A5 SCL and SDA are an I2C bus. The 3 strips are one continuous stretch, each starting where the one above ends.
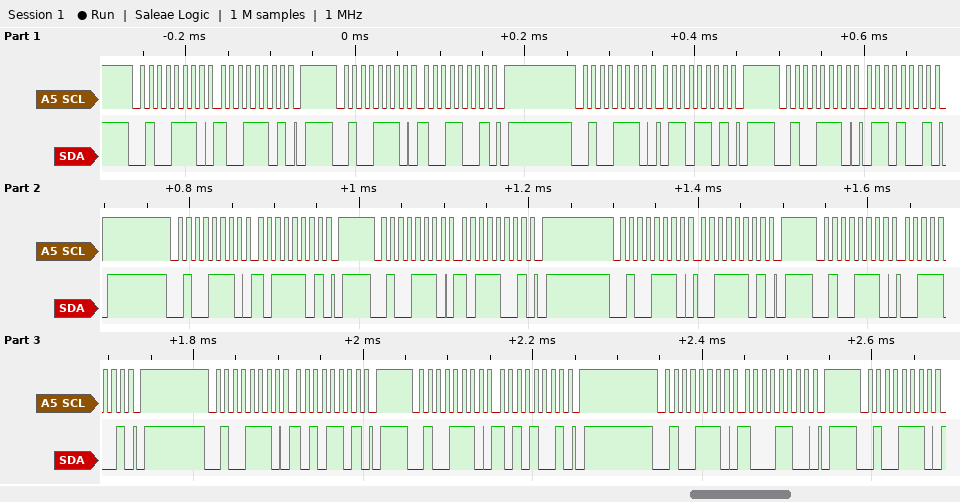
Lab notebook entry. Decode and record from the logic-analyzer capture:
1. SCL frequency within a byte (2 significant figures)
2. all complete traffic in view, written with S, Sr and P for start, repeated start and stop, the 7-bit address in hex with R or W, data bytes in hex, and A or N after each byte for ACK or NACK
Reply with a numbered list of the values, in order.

1. 100 kHz
2. S 27W A 9D A P S 27W A 99 A P S 27W A 6D A P S 27W A 69 A P S 27W A BD A P S 27W A B9 A P S 27W A 3D A P S 27W A 39 A P S 27W A AD A P S 27W A A9 A P S 27W A 8C A P S 27W A
